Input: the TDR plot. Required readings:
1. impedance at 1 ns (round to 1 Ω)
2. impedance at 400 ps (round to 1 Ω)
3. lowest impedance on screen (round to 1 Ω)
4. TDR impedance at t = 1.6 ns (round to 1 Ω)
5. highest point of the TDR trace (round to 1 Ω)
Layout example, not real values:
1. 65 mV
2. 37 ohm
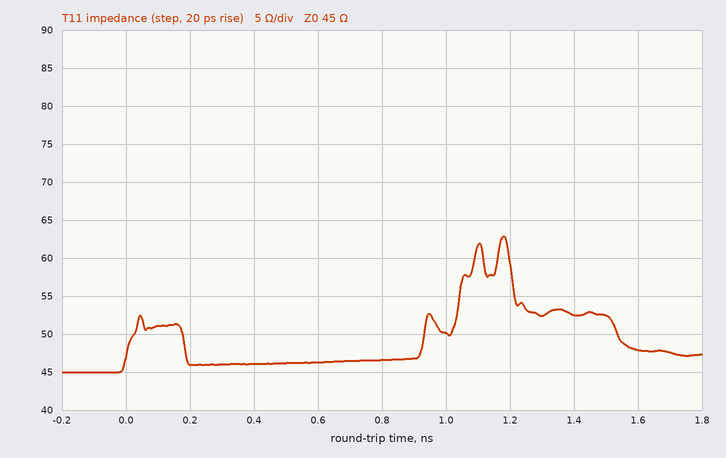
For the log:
1. 50 Ω
2. 46 Ω
3. 45 Ω
4. 48 Ω
5. 63 Ω
